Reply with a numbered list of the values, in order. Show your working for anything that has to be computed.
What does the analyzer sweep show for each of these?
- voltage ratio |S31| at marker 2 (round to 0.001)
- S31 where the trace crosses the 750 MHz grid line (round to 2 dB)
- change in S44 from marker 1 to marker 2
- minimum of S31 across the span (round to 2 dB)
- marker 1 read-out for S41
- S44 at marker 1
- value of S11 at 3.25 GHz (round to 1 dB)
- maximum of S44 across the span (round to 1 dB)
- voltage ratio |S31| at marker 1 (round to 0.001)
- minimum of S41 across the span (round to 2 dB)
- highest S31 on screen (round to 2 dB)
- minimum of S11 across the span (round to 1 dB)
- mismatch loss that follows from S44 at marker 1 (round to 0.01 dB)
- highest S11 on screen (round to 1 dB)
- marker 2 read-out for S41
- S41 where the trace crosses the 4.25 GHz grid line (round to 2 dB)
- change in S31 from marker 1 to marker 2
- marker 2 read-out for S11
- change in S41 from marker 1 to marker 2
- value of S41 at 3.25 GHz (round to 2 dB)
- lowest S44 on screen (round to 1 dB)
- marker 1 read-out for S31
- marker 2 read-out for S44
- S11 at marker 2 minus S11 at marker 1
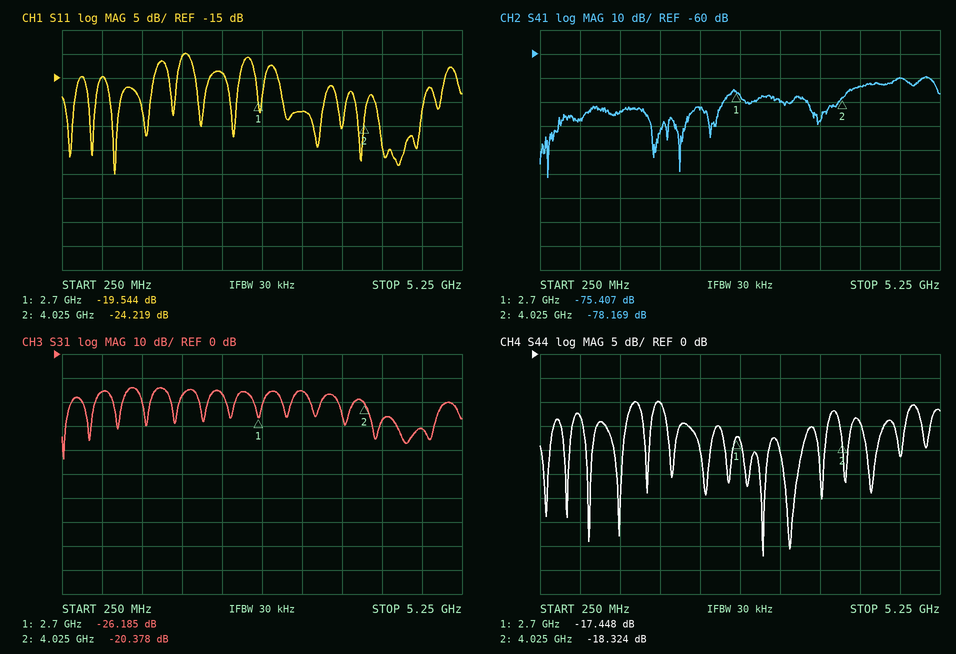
1. 10^(-20.378/20) ≈ 0.096
2. -16 dB
3. -18.324 − (-17.448) = -0.876 dB
4. -44 dB
5. -75.407 dB
6. -17.448 dB
7. -22 dB
8. -10 dB
9. 10^(-26.185/20) ≈ 0.049
10. -112 dB
11. -14 dB
12. -35 dB
13. −10 log10(1 − 10^(-17.448/10)) ≈ 0.08 dB
14. -10 dB
15. -78.169 dB
16. -74 dB
17. -20.378 − (-26.185) = 5.807 dB
18. -24.219 dB
19. -78.169 − (-75.407) = -2.762 dB
20. -80 dB
21. -42 dB
22. -26.185 dB
23. -18.324 dB
24. -24.219 − (-19.544) = -4.675 dB
